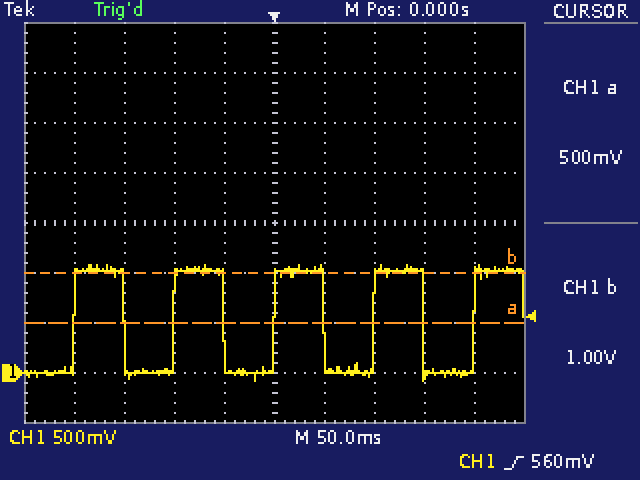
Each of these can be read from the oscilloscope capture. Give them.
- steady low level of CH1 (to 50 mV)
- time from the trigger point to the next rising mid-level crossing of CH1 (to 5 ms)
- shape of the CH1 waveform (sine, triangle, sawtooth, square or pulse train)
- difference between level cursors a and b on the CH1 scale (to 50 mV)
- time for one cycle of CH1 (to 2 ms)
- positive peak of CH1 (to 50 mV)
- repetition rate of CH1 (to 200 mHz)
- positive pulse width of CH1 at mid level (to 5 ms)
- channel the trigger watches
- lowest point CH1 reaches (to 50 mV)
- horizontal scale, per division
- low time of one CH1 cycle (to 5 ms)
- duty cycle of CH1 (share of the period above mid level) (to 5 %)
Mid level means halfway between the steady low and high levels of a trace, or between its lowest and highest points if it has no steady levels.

0 mV
100 ms
square
500 mV
100 ms
1.10 V
10.0 Hz
50 ms
CH1
-100 mV
50 ms
50 ms
50 %
